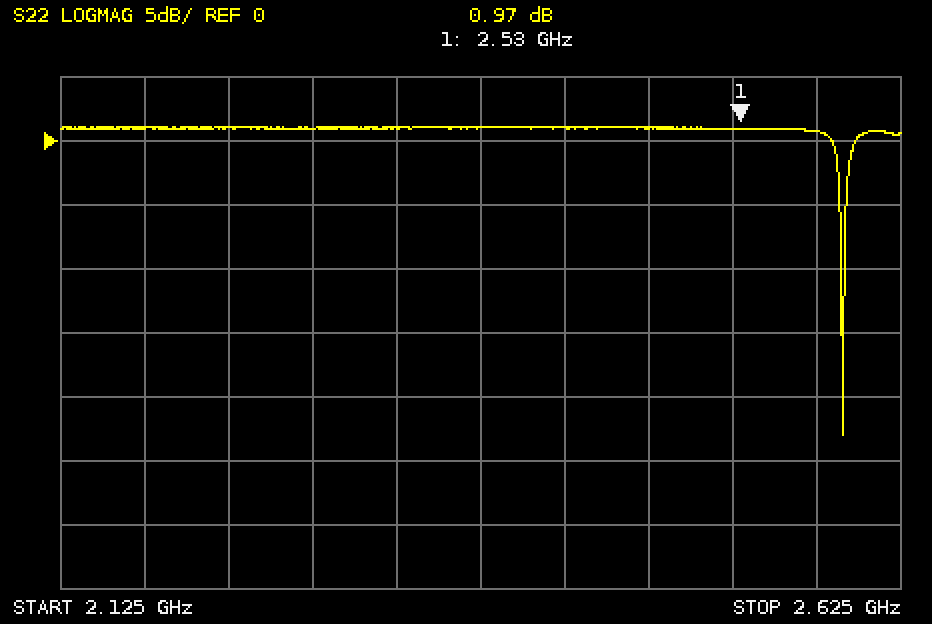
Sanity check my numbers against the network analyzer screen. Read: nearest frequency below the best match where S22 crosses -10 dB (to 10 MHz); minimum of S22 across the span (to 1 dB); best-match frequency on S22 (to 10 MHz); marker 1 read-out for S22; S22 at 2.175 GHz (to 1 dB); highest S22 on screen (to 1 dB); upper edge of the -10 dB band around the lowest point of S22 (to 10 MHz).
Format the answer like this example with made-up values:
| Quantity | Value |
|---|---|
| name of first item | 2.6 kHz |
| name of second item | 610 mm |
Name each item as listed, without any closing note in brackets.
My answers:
| Quantity | Value |
|---|---|
| nearest frequency below the best match where S22 crosses -10 dB | 2.59 GHz |
| minimum of S22 across the span | -23 dB |
| best-match frequency on S22 | 2.59 GHz |
| marker 1 read-out for S22 | 0.97 dB |
| S22 at 2.175 GHz | 1 dB |
| highest S22 on screen | 1 dB |
| upper edge of the -10 dB band around the lowest point of S22 | 2.59 GHz |
